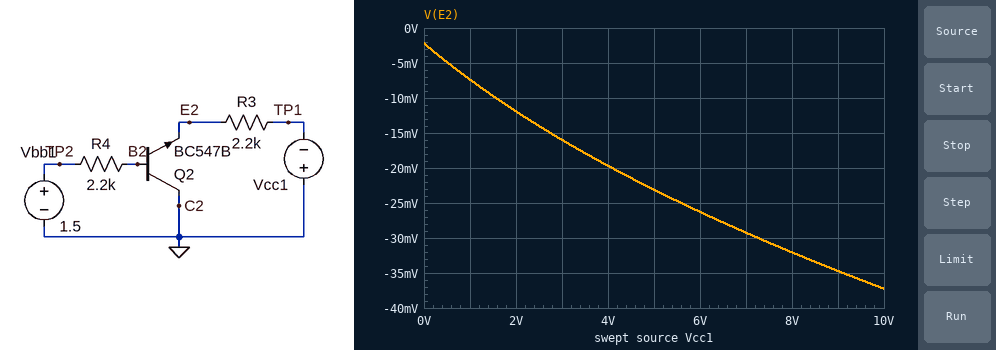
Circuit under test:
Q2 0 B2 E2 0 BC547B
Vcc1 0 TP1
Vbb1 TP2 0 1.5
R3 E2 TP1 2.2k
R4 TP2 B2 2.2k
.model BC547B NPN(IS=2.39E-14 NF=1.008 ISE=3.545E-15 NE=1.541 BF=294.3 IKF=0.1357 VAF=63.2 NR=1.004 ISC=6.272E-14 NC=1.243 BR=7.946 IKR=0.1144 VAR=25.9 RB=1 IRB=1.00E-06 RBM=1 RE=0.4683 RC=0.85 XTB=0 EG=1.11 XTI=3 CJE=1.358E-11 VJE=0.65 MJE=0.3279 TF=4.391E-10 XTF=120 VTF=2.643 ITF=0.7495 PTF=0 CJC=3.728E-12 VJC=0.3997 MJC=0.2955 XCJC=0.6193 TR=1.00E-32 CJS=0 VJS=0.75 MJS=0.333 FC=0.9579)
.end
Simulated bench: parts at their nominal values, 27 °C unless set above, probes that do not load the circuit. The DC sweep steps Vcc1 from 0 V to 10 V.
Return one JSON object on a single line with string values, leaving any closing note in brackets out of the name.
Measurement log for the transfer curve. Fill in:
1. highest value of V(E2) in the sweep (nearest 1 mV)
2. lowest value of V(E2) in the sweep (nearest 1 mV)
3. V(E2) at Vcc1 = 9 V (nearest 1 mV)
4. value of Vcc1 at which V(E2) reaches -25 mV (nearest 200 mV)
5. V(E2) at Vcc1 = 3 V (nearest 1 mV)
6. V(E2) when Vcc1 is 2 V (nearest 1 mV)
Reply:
{"highest value of V(E2) in the sweep": "-2 mV", "lowest value of V(E2) in the sweep": "-37 mV", "V(E2) at Vcc1 = 9 V": "-35 mV", "value of Vcc1 at which V(E2) reaches -25 mV": "5.6 V", "V(E2) at Vcc1 = 3 V": "-16 mV", "V(E2) when Vcc1 is 2 V": "-12 mV"}
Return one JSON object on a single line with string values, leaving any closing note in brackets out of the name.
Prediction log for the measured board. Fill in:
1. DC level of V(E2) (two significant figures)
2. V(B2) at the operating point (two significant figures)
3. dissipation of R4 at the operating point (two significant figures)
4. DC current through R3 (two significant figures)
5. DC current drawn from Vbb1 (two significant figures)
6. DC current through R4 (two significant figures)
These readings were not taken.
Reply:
{"DC level of V(E2)": "-2.2 mV", "V(B2) at the operating point": "660 mV", "dissipation of R4 at the operating point": "320 µW", "DC current through R3": "1.0 µA", "DC current drawn from Vbb1": "380 µA", "DC current through R4": "380 µA"}
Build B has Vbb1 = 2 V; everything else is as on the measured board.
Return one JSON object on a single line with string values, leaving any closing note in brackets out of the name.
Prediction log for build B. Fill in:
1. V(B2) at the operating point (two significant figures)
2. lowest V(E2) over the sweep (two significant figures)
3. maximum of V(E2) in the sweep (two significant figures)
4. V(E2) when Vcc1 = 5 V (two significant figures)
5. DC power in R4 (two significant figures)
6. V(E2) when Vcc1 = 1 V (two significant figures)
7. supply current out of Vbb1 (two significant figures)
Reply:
{"V(B2) at the operating point": "670 mV", "lowest V(E2) over the sweep": "-30 mV", "maximum of V(E2) in the sweep": "-2.1 mV", "V(E2) when Vcc1 = 5 V": "-18 mV", "DC power in R4": "800 µW", "V(E2) when Vcc1 = 1 V": "-5.7 mV", "supply current out of Vbb1": "600 µA"}
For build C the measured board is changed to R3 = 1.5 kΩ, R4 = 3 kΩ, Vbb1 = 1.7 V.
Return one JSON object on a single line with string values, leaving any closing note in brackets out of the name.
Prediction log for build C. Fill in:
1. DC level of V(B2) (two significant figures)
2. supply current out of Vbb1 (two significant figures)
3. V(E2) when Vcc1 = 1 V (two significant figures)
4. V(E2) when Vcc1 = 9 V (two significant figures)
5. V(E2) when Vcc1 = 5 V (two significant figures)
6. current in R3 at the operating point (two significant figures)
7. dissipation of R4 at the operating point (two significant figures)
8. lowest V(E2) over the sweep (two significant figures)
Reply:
{"DC level of V(B2)": "660 mV", "supply current out of Vbb1": "350 µA", "V(E2) when Vcc1 = 1 V": "-10 mV", "V(E2) when Vcc1 = 9 V": "-47 mV", "V(E2) when Vcc1 = 5 V": "-32 mV", "current in R3 at the operating point": "1.5 µA", "dissipation of R4 at the operating point": "360 µW", "lowest V(E2) over the sweep": "-50 mV"}
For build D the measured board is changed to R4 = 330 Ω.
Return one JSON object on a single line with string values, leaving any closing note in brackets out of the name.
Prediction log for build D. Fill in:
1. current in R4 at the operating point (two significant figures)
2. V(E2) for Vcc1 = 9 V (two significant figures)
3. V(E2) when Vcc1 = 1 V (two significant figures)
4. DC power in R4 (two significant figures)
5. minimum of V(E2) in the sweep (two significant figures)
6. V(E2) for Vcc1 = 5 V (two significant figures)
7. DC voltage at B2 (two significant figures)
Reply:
{"current in R4 at the operating point": "2.4 mA", "V(E2) for Vcc1 = 9 V": "-13 mV", "V(E2) when Vcc1 = 1 V": "-2.2 mV", "DC power in R4": "1.9 mW", "minimum of V(E2) in the sweep": "-15 mV", "V(E2) for Vcc1 = 5 V": "-7.9 mV", "DC voltage at B2": "710 mV"}
